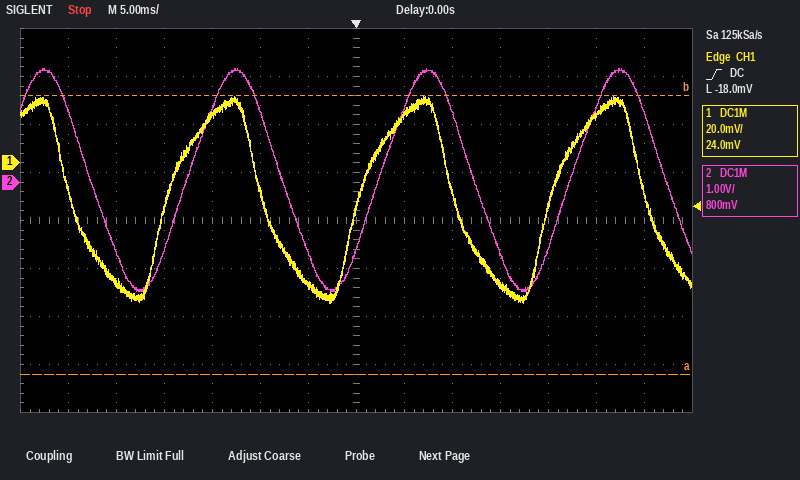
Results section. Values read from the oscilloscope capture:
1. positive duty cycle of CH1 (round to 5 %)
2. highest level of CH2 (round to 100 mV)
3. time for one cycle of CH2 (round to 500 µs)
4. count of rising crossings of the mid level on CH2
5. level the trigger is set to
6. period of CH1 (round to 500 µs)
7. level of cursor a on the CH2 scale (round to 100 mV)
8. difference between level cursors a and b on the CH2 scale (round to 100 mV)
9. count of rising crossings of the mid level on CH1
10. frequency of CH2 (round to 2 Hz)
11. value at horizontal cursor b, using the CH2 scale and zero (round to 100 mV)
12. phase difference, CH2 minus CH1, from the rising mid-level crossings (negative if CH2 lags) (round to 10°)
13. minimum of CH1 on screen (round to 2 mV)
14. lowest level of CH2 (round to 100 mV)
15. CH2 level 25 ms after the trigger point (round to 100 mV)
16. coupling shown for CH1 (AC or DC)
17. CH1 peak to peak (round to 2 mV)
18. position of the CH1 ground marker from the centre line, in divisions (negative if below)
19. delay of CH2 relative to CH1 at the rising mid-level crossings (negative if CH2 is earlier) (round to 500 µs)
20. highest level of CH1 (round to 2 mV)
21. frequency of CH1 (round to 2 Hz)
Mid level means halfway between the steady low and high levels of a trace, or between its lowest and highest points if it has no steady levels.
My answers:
50 %
2.4 V
20.0 ms
3
-18.0 mV
20.0 ms
-4.0 V
5.8 V
3
50 Hz
1.8 V
-40°
-58 mV
-2.3 V
1.5 V
DC
86 mV
+1.2 div
+2.0 ms
28 mV
50 Hz
